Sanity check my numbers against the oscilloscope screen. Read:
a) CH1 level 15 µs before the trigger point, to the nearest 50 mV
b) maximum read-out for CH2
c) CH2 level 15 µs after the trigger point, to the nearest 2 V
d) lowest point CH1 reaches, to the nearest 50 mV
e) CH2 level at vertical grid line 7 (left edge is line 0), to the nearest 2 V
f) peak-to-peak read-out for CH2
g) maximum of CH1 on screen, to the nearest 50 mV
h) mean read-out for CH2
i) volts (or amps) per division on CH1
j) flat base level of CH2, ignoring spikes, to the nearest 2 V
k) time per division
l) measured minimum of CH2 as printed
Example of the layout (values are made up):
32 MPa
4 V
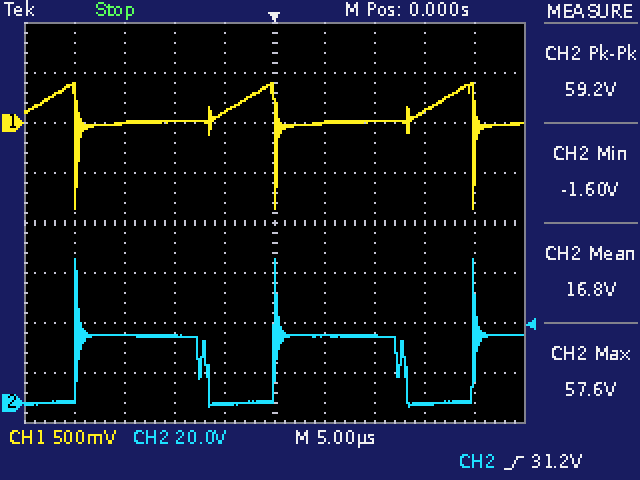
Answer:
0 mV
57.6 V
0 V
-850 mV
26 V
59.2 V
400 mV
16.8 V
500 mV
0 V
5 µs
-1.60 V
